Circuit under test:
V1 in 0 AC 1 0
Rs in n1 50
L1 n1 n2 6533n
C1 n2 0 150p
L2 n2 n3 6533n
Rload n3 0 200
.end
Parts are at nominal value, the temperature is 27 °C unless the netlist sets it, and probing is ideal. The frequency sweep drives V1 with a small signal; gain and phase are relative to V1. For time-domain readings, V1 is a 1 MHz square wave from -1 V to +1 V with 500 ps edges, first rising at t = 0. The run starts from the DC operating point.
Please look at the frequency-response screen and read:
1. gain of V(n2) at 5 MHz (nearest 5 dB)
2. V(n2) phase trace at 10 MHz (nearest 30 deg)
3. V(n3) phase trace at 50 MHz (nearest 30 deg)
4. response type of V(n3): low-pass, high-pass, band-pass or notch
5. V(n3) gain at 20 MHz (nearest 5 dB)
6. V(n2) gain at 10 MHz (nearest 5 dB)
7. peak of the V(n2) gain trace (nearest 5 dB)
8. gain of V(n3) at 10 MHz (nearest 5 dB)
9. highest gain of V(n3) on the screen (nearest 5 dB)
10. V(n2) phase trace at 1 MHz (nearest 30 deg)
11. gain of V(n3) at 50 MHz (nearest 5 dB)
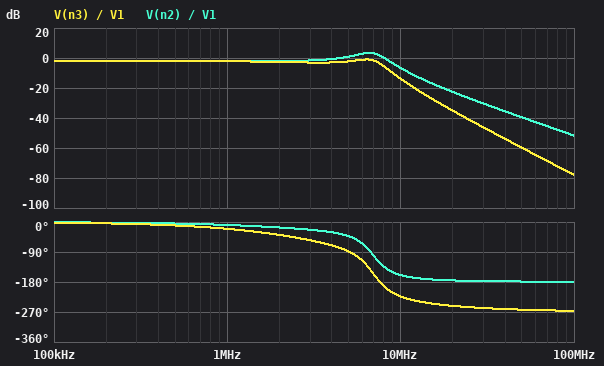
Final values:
0 dB
-150 deg
-270 deg
low-pass
-35 dB
-5 dB
5 dB
-15 dB
0 dB
0 deg
-60 dB
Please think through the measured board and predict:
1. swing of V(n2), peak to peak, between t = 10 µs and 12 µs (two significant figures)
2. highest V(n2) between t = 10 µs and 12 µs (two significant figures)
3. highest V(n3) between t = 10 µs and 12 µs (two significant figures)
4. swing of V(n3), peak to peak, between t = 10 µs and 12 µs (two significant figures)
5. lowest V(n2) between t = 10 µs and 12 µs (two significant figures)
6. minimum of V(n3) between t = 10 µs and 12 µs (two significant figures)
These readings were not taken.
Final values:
2.6 V
1.3 V
920 mV
1.8 V
-1.3 V
-920 mV
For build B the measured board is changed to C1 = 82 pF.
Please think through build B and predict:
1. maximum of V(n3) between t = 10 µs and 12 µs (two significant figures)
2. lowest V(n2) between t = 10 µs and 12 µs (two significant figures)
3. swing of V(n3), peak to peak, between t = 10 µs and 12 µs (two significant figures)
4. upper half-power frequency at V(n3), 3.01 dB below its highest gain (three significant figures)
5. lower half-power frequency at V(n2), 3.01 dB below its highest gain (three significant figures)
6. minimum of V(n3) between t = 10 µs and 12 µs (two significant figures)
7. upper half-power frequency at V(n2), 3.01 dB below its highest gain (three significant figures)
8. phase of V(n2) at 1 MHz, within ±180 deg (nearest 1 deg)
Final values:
860 mV
-1.3 V
1.7 V
10.4 MHz
7.60 MHz
-860 mV
10.7 MHz
-8 deg
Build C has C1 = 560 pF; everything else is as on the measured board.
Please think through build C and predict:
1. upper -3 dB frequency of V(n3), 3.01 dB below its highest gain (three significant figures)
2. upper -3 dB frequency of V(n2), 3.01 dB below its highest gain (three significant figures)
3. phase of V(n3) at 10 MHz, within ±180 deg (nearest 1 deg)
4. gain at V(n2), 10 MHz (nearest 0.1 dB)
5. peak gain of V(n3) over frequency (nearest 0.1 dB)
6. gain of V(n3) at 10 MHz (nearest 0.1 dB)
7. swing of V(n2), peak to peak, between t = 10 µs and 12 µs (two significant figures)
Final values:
3.73 MHz
3.89 MHz
125 deg
-22.1 dB
0 dB
-29.3 dB
2.5 V
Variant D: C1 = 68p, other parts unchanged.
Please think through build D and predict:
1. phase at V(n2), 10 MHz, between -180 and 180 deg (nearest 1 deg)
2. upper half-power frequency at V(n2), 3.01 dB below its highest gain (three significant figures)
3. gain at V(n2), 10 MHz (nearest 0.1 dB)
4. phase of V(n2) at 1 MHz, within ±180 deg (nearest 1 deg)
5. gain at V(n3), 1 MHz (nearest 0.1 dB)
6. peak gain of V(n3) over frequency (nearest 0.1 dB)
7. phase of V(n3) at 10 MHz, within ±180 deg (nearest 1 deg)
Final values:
-79 deg
11.7 MHz
5.7 dB
-8 deg
-2.3 dB
-1.5 dB
-143 deg
